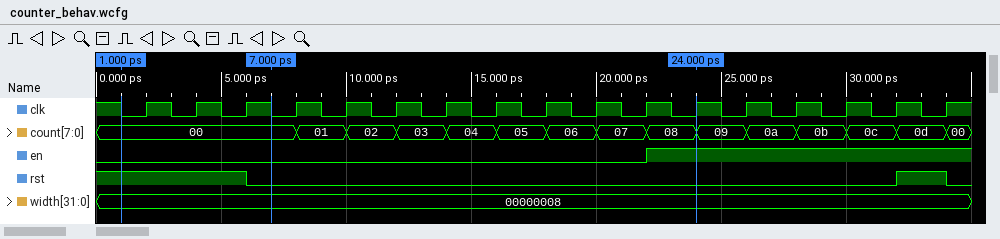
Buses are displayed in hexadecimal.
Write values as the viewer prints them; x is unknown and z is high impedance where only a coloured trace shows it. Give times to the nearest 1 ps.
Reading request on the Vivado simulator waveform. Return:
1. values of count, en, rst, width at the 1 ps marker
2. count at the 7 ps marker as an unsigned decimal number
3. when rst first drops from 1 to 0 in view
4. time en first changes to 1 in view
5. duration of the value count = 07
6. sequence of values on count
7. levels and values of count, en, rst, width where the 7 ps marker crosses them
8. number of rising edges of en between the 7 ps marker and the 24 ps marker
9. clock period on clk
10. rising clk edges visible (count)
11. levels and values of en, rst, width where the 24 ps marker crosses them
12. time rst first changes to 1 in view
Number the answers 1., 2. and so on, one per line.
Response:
1. count=00, en=0, rst=1, width=00000008
2. 0
3. 6 ps
4. 22 ps
5. 2 ps
6. 00, 01, 02, 03, 04, 05, 06, 07, 08, 09, 0a, 0b, 0c, 0d, 00
7. count=00, en=0, rst=0, width=00000008
8. 1
9. 2 ps
10. 17
11. en=1, rst=0, width=00000008
12. 32 ps
